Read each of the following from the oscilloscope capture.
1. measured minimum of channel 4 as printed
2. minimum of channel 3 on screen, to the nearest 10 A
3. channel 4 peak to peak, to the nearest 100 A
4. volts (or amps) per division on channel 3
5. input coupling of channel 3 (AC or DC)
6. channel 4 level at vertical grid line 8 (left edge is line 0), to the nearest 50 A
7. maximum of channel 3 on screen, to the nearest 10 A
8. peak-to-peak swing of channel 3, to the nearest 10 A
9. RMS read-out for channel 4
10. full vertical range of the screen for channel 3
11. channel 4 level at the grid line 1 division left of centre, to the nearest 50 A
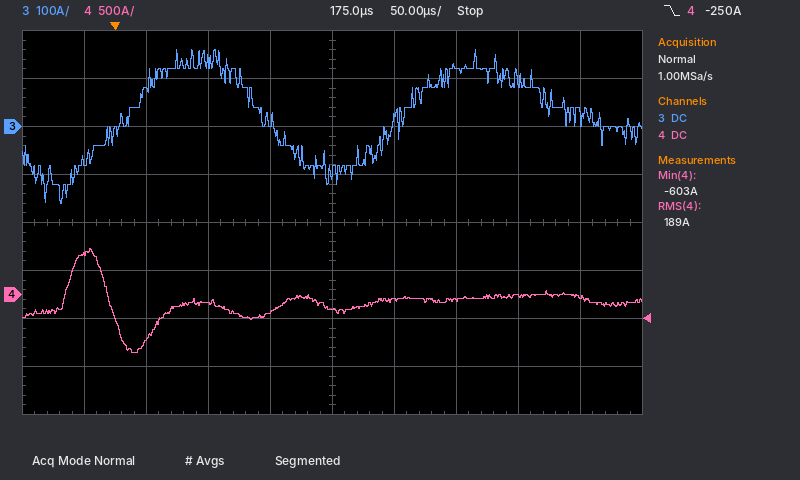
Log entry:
-603 A
-160 A
1.10 kA
100 A
DC
0 A
160 A
320 A
189 A
800 A
-200 A
